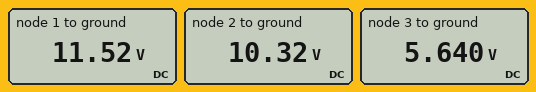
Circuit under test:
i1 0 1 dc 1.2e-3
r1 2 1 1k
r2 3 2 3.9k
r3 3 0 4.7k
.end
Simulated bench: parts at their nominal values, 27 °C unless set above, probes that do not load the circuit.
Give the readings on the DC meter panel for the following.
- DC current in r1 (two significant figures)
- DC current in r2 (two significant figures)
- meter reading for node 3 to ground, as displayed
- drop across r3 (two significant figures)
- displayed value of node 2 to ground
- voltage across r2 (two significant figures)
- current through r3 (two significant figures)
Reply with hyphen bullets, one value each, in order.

- 1.2 mA
- 1.2 mA
- 5.640 V
- 5.6 V
- 10.32 V
- 4.7 V
- 1.2 mA
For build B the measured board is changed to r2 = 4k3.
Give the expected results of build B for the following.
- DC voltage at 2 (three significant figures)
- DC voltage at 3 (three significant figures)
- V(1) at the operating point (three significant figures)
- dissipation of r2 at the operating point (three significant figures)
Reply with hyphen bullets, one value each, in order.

- 10.8 V
- 5.64 V
- 12.0 V
- 6.19 mW
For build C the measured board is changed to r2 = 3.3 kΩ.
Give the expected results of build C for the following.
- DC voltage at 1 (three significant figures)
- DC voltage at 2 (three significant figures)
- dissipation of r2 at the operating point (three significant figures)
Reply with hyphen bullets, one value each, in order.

- 10.8 V
- 9.60 V
- 4.75 mW
